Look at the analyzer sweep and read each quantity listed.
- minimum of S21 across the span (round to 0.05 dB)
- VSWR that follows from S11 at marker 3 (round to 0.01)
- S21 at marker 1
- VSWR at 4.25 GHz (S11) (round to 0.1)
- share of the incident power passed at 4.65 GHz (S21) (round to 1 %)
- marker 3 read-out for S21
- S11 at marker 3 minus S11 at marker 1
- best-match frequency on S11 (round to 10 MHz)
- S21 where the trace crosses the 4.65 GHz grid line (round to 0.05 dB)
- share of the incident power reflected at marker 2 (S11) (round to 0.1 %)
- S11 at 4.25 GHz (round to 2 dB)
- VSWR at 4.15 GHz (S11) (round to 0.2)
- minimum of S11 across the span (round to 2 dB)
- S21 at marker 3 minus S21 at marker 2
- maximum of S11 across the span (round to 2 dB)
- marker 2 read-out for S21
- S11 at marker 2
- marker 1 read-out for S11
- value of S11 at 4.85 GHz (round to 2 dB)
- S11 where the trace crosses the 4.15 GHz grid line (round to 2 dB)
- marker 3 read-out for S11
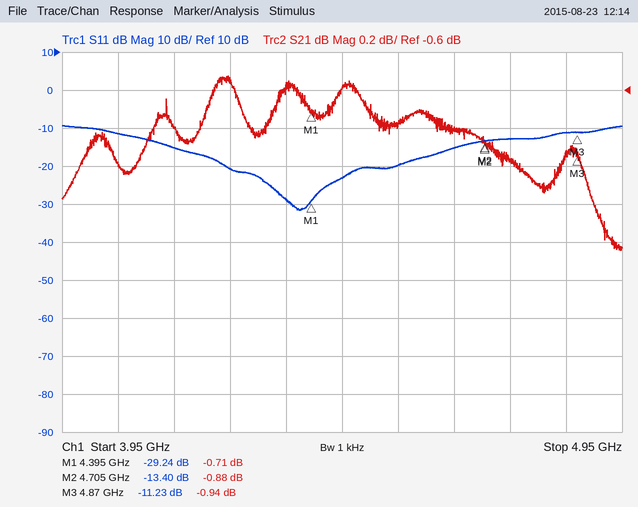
-1.45 dB
1.76
-0.71 dB
1.2
83 %
-0.94 dB
18.01 dB
4.37 GHz
-0.80 dB
4.6 %
-20 dB
1.4
-32 dB
-0.06 dB
-10 dB
-0.88 dB
-13.40 dB
-29.24 dB
-12 dB
-16 dB
-11.23 dB
